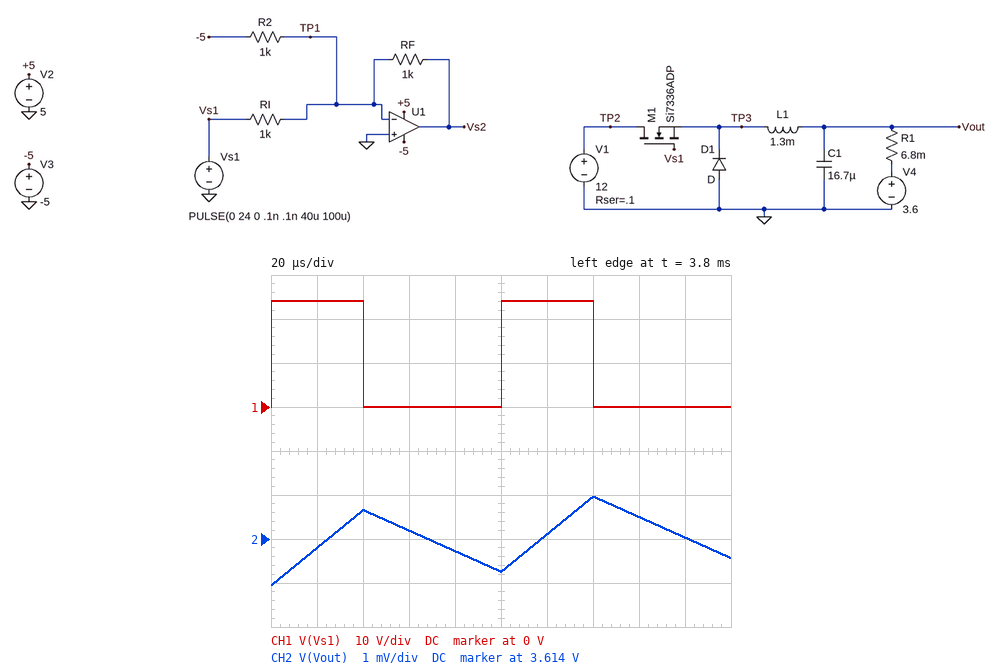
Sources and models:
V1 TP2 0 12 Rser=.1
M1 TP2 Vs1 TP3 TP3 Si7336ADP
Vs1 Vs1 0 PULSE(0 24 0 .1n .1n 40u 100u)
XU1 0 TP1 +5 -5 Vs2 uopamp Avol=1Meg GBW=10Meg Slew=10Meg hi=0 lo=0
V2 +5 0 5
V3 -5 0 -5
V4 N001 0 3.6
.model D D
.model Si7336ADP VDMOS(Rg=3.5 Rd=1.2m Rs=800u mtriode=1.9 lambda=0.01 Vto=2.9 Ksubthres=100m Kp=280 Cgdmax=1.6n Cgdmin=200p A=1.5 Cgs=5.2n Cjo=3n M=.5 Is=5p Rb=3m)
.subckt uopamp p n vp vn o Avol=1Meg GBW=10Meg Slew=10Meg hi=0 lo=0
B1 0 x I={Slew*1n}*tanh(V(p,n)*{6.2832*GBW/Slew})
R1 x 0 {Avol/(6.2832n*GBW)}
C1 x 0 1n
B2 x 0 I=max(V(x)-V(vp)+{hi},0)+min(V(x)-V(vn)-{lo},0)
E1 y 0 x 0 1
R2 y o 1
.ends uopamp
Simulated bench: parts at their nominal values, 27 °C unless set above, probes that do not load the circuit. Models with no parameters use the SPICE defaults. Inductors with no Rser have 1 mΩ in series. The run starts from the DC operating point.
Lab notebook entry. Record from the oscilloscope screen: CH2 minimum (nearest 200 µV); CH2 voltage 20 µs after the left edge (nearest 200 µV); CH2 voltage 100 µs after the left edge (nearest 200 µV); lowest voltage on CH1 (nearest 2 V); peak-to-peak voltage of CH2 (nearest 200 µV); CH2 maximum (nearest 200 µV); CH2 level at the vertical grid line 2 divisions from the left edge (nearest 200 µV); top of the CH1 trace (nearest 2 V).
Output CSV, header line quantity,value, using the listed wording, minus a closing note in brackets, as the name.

quantity,value
CH2 minimum,3.6130 V
CH2 voltage 20 µs after the left edge,3.6138 V
CH2 voltage 100 µs after the left edge,3.6132 V
lowest voltage on CH1,0 V
peak-to-peak voltage of CH2,2.0 mV
CH2 maximum,3.6150 V
CH2 level at the vertical grid line 2 divisions from the left edge,3.6146 V
top of the CH1 trace,24 V
